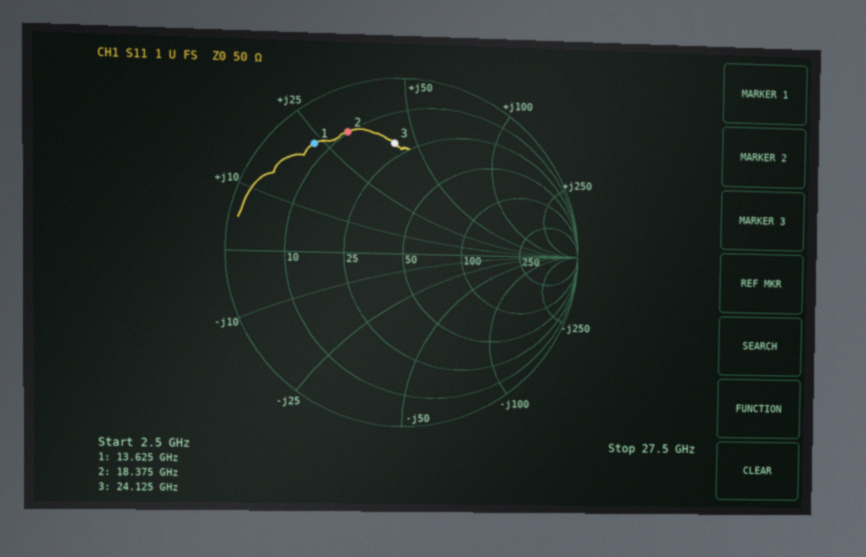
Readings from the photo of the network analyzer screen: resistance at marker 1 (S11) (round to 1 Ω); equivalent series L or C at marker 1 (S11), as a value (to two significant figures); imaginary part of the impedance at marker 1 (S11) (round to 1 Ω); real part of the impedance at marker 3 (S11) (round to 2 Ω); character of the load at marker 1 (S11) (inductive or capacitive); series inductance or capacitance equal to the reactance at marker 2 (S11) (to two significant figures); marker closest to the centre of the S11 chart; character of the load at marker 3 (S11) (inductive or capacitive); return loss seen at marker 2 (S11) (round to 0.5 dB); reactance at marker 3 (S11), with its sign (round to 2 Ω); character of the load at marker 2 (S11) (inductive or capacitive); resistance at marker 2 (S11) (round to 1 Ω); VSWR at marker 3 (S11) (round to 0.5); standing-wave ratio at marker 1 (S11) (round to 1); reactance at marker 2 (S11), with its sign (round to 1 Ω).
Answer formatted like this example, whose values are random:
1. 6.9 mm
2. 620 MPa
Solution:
1. 7 Ω
2. 270 pH
3. +23 Ω
4. 20 Ω
5. inductive
6. 270 pH
7. marker 3
8. inductive
9. 2.5 dB
10. +42 Ω
11. inductive
12. 10 Ω
13. 4.5
14. 9
15. +31 Ω
